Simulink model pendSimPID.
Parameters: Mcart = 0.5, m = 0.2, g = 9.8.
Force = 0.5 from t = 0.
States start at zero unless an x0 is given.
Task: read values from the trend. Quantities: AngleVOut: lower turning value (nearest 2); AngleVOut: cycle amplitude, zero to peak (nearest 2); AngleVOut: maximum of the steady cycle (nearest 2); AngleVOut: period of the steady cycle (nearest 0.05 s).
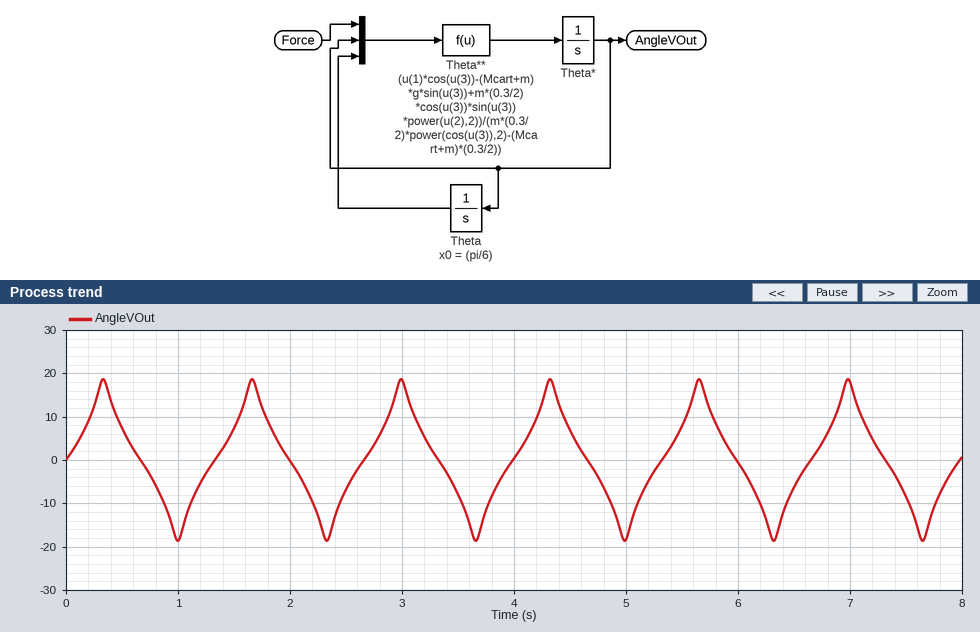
-18
18
18
1.35 s
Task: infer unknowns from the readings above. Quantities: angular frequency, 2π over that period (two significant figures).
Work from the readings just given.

4.7 rad/s
